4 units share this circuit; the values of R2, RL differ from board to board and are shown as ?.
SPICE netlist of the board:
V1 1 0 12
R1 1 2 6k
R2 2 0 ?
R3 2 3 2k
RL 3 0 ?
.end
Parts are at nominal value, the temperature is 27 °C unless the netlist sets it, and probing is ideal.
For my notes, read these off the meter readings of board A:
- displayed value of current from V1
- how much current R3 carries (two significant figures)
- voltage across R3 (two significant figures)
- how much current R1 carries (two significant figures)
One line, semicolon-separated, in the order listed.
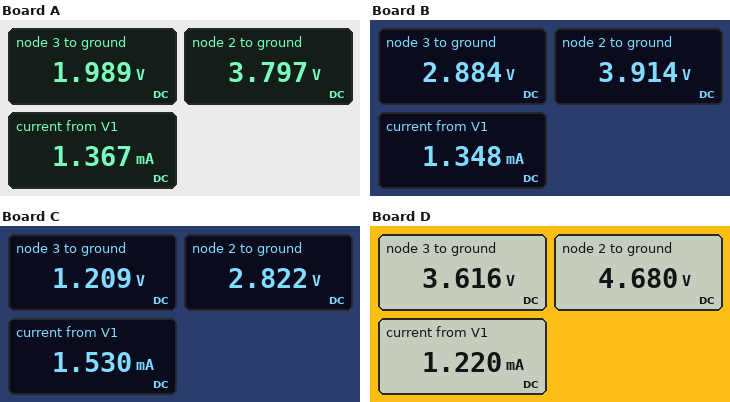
1.367 mA; 900 µA; 1.8 V; 1.4 mA
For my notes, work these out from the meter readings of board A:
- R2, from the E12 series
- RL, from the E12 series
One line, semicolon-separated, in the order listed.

8.2 kΩ; 2.2 kΩ
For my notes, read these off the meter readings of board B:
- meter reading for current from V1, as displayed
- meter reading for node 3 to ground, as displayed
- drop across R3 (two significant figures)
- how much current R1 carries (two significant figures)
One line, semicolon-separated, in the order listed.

1.348 mA; 2.884 V; 1.0 V; 1.3 mA
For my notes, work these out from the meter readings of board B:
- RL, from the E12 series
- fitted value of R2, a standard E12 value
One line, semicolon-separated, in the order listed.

5.6 kΩ; 4.7 kΩ
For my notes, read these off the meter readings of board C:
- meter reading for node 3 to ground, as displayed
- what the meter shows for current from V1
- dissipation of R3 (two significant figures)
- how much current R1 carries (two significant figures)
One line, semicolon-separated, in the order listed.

1.209 V; 1.530 mA; 1.3 mW; 1.5 mA
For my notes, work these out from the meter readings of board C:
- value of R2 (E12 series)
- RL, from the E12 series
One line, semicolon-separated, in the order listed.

3.9 kΩ; 1.5 kΩ
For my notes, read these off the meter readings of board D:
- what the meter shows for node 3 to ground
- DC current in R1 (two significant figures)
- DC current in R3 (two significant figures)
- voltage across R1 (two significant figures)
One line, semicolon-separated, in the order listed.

3.616 V; 1.2 mA; 530 µA; 7.3 V
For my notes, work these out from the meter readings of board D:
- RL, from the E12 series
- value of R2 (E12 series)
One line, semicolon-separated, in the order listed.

6.8 kΩ; 6.8 kΩ
